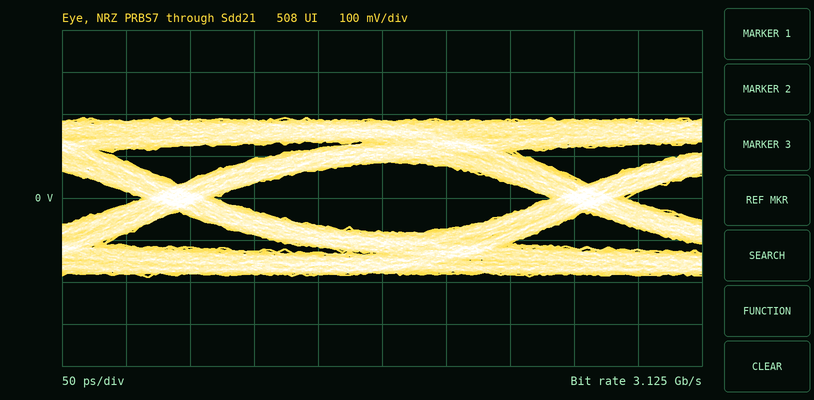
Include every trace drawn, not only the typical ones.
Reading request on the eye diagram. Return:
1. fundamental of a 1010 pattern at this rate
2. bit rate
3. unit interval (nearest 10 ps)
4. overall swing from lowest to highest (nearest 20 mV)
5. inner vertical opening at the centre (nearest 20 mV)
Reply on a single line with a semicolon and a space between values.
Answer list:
1.5625 GHz; 3.125 Gb/s; 320 ps; 380 mV; 160 mV
